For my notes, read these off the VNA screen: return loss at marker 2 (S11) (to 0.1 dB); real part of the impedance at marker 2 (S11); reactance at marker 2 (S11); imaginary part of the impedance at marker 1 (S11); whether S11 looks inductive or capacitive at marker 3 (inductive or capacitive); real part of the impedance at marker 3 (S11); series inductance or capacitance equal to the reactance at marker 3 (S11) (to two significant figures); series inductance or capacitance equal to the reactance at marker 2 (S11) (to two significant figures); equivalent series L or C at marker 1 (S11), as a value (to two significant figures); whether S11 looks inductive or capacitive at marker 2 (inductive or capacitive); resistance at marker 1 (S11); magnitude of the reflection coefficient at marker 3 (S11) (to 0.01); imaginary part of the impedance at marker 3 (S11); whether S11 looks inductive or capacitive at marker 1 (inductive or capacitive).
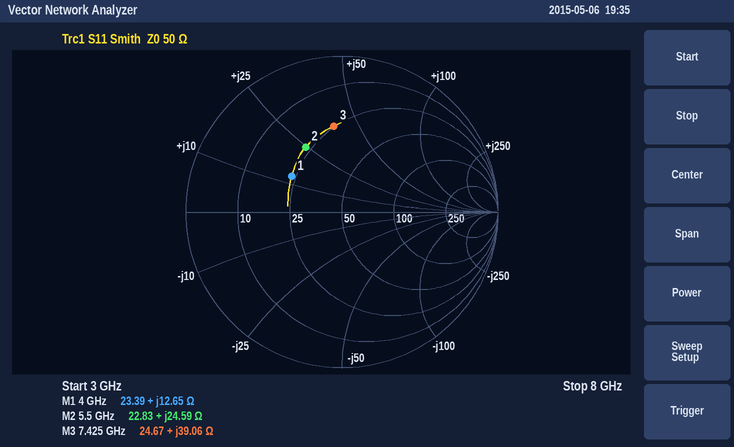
6.4 dB
22.83 Ω
+24.59 Ω
+12.65 Ω
inductive
24.67 Ω
840 pH
710 pH
500 pH
inductive
23.39 Ω
0.55
+39.06 Ω
inductive
